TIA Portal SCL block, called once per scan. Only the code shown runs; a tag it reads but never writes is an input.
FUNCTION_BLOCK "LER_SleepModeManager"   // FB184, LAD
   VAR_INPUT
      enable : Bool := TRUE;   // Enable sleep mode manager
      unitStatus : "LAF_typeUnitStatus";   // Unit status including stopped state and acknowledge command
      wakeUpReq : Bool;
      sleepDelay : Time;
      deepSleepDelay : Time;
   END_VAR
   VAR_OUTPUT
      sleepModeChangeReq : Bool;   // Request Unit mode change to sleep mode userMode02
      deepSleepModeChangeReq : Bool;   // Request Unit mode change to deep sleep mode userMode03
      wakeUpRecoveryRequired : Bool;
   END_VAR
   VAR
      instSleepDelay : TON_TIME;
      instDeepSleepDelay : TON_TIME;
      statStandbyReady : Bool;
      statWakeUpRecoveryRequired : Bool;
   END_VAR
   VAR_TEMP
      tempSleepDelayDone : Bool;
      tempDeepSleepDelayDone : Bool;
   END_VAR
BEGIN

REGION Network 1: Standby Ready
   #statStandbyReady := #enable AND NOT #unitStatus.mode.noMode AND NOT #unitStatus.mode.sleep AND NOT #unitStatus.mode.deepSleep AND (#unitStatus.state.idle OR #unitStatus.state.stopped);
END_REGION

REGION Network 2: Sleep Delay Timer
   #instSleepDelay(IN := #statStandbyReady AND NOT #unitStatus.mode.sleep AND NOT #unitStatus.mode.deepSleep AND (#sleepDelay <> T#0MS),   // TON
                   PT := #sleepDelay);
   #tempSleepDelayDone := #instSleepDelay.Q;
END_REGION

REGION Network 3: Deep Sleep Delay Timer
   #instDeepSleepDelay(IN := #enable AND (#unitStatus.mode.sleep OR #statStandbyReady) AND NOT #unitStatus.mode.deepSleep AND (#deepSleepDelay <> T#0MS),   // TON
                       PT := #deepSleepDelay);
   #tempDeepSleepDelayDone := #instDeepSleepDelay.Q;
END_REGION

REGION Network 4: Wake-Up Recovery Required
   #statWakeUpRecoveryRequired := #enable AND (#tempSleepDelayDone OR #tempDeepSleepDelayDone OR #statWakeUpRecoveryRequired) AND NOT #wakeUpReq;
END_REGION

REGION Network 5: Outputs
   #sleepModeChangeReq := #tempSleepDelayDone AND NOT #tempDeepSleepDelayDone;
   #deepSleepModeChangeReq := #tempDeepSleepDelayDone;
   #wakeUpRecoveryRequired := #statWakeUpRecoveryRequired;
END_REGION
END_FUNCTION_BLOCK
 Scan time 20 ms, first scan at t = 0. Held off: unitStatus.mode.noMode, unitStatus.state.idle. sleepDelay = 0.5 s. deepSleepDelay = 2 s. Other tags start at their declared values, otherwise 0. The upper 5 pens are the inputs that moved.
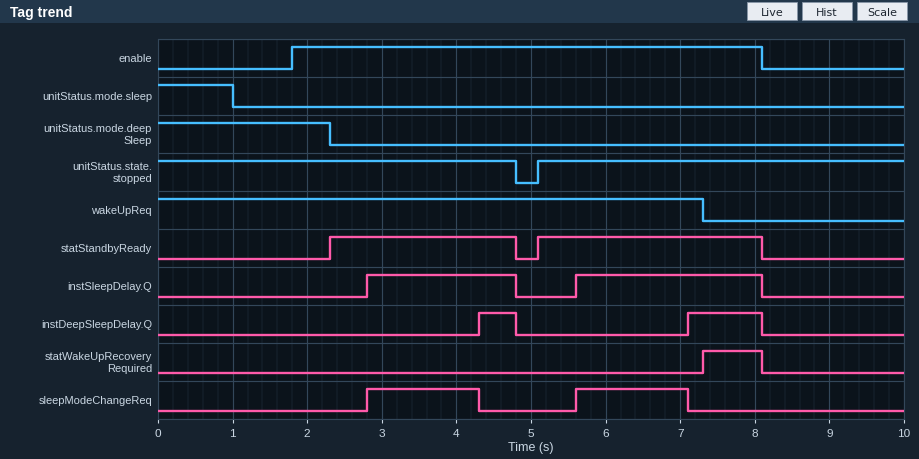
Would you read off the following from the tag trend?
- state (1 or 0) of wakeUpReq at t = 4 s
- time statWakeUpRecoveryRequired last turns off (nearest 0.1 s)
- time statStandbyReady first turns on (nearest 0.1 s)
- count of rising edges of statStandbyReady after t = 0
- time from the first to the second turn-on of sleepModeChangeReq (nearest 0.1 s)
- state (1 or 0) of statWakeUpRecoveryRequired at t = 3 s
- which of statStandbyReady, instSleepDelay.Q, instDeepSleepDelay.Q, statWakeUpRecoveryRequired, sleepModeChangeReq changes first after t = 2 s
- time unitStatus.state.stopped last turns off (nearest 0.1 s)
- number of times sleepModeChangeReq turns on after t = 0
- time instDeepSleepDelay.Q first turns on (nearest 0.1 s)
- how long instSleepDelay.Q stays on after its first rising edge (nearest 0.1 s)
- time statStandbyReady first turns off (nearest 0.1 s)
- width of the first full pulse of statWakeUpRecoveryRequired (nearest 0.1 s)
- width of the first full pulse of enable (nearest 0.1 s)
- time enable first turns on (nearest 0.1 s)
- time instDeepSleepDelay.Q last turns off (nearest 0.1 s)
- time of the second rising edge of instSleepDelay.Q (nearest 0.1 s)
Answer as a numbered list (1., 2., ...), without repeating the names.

1. 1
2. 8.1 s
3. 2.3 s
4. 2
5. 2.8 s
6. 0
7. statStandbyReady
8. 4.8 s
9. 2
10. 4.3 s
11. 2.0 s
12. 4.8 s
13. 0.8 s
14. 6.3 s
15. 1.8 s
16. 8.1 s
17. 5.6 s
